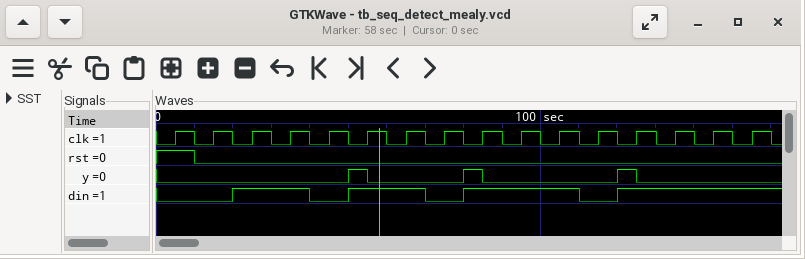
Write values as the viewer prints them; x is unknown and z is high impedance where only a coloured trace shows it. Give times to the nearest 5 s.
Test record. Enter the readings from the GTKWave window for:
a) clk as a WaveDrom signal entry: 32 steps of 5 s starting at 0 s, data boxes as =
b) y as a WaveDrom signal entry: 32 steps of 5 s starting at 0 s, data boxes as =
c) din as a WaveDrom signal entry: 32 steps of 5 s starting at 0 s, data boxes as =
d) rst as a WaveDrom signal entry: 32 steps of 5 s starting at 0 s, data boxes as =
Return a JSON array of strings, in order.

["{name: 'clk', wave: '01010101010101010101010101010101'}", "{name: 'y', wave: '0.........10....10......10......'}", "{name: 'din', wave: '0...1...0.1...0.1.....0.1.......'}", "{name: 'rst', wave: '1.0.............................'}"]
